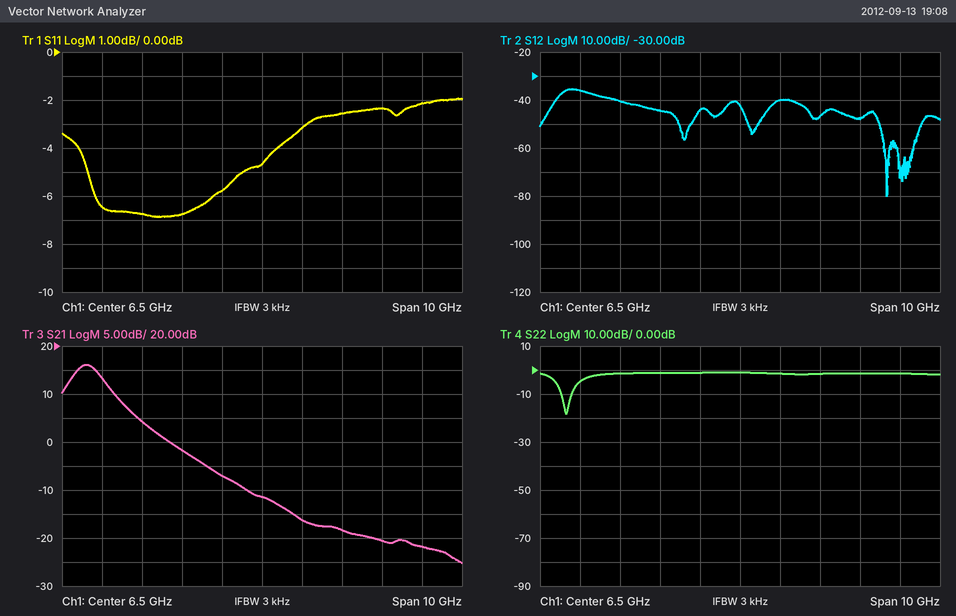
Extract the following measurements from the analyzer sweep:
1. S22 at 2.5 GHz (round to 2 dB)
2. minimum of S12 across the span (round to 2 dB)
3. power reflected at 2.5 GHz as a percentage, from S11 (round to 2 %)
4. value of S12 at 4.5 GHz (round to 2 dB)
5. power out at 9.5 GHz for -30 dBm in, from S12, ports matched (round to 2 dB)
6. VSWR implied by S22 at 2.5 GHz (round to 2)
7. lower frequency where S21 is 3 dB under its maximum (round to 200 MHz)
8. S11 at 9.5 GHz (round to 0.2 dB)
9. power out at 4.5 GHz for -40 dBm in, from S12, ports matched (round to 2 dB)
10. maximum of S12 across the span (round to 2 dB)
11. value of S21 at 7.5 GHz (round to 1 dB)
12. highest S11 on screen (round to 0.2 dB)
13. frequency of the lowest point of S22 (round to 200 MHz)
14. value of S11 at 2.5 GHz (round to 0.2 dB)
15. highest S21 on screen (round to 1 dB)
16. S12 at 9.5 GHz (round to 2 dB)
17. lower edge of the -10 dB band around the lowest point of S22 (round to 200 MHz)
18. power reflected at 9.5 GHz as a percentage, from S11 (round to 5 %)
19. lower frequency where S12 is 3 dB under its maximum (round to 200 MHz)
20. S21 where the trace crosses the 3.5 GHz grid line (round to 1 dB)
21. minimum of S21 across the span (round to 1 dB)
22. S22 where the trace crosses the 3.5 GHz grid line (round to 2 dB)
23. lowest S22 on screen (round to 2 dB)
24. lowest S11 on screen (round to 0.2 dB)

-4 dB
-80 dB
22 %
-44 dB
-78 dBm
4
1.8 GHz
-2.4 dB
-84 dBm
-36 dB
-16 dB
-2.0 dB
2.2 GHz
-6.4 dB
16 dB
-48 dB
2.0 GHz
60 %
2.0 GHz
4 dB
-25 dB
-2 dB
-18 dB
-6.8 dB
